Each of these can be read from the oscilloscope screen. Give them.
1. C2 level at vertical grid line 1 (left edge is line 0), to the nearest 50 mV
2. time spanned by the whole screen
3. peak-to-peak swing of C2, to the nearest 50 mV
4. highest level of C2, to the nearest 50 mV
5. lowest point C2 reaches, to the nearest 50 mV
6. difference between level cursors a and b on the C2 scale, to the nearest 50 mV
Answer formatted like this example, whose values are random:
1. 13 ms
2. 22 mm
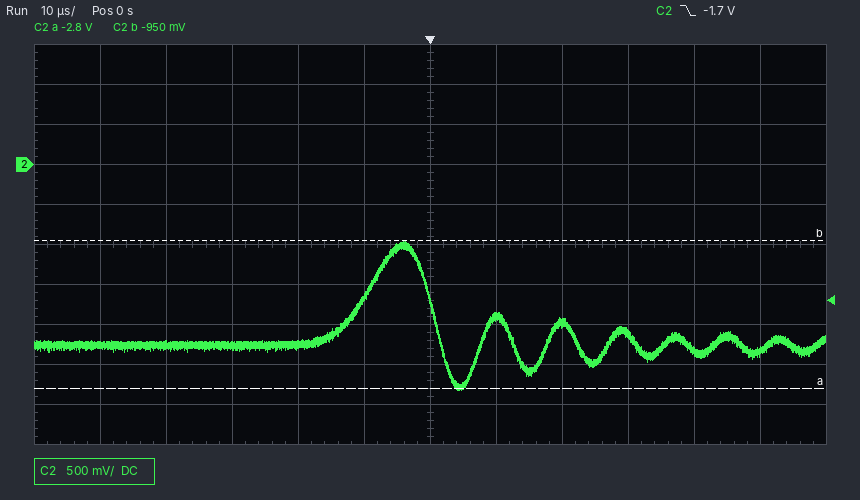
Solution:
1. -2.25 V
2. 120 µs
3. 1.85 V
4. -950 mV
5. -2.80 V
6. 1.85 V
